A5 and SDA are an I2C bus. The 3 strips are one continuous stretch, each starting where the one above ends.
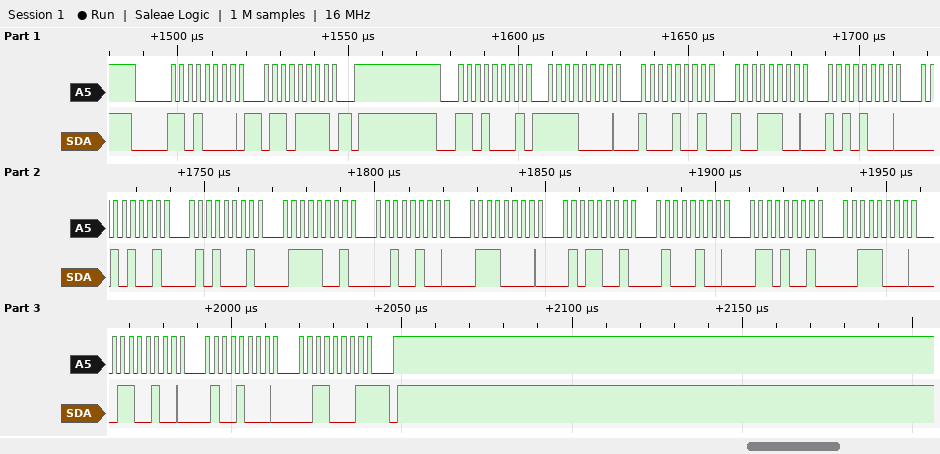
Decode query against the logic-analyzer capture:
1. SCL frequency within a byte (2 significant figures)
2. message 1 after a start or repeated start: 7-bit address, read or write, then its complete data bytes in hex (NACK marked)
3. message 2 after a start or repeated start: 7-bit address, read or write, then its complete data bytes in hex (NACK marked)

400 kHz
0x68 write: 6F
0x68 read: F0 89 9C A8 29 51 79 24 70 59 44 69 38 64 48 31 NACK
